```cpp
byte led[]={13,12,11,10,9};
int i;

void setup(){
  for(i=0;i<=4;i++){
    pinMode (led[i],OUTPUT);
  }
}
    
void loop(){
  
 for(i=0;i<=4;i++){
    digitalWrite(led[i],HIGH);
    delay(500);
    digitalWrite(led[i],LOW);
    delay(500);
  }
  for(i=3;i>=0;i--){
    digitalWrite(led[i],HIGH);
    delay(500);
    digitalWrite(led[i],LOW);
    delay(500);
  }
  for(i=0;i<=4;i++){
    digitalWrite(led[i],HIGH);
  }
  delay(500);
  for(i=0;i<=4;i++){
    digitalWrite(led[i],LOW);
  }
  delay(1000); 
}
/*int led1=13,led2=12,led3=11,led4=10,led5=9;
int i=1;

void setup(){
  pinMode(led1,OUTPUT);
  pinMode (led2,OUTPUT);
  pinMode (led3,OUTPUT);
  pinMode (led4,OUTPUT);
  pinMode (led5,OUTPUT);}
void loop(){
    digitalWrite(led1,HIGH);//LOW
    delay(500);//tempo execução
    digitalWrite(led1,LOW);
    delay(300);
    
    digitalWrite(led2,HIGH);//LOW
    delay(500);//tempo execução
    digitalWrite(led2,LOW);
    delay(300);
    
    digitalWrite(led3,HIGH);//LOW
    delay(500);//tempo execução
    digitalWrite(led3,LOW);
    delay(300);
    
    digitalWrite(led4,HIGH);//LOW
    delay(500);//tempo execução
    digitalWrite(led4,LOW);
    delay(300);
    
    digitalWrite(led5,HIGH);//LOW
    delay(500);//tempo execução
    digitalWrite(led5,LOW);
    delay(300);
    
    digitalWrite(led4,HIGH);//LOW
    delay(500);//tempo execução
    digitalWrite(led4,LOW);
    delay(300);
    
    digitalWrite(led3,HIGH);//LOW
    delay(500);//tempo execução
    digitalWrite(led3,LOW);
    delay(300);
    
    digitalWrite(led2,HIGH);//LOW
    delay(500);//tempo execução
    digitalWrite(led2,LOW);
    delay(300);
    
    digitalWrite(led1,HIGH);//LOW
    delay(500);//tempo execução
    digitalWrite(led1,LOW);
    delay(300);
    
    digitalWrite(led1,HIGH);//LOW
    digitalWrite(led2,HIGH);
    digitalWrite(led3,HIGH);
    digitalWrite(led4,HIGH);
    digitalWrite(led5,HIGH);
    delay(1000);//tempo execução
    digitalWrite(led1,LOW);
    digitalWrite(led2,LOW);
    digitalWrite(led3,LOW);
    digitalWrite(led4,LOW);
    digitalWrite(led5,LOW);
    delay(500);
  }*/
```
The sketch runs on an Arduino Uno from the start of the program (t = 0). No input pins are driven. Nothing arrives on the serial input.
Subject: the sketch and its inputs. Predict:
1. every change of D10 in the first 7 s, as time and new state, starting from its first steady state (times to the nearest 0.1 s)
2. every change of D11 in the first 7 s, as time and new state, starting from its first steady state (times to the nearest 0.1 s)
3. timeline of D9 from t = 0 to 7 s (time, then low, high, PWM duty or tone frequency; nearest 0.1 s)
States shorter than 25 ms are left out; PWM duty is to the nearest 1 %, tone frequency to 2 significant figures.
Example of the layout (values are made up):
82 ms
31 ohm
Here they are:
0 s low; 3 s high; 3.5 s low; 5 s high; 5.5 s low
0 s low; 2 s high; 2.5 s low; 6 s high; 6.5 s low
0 s low; 4 s high; 4.5 s low
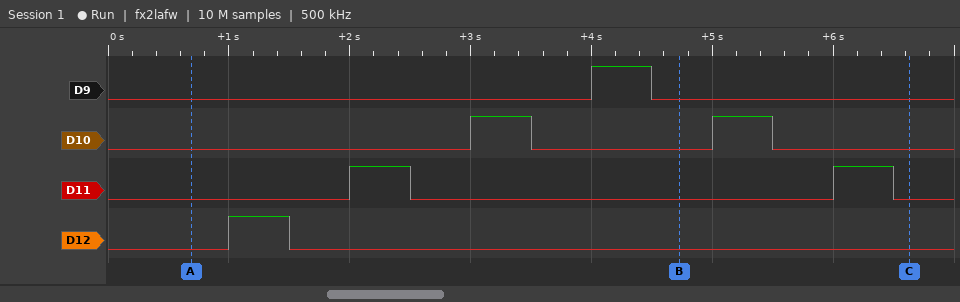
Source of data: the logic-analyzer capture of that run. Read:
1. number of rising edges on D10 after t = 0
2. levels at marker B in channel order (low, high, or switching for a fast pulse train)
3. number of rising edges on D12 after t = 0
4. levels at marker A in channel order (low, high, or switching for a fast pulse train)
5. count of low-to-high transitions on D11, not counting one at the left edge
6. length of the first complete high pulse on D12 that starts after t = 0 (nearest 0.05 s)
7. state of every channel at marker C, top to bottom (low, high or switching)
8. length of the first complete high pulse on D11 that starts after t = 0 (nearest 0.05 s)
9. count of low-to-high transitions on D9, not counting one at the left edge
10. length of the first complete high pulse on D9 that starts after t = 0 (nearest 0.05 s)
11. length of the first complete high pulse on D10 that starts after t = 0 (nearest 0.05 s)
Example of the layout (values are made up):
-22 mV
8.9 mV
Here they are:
2
D9 low, D10 low, D11 low, D12 low
1
D9 low, D10 low, D11 low, D12 low
2
0.50 s
D9 low, D10 low, D11 low, D12 low
0.50 s
1
0.50 s
0.50 s
